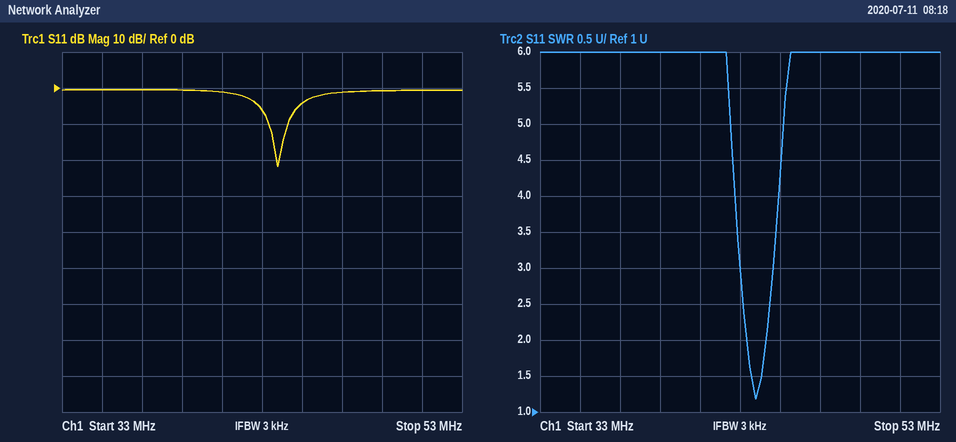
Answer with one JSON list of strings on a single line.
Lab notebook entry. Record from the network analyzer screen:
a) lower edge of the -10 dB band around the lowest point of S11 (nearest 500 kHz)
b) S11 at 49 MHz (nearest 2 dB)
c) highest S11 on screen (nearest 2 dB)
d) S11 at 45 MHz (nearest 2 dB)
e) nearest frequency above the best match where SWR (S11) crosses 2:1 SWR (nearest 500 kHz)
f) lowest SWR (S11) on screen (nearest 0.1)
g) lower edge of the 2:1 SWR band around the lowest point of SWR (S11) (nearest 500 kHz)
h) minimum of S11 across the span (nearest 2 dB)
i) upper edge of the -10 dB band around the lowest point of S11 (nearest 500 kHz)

["43.5 MHz", "0 dB", "0 dB", "-4 dB", "44.5 MHz", "1.2", "43.5 MHz", "-22 dB", "44.5 MHz"]
